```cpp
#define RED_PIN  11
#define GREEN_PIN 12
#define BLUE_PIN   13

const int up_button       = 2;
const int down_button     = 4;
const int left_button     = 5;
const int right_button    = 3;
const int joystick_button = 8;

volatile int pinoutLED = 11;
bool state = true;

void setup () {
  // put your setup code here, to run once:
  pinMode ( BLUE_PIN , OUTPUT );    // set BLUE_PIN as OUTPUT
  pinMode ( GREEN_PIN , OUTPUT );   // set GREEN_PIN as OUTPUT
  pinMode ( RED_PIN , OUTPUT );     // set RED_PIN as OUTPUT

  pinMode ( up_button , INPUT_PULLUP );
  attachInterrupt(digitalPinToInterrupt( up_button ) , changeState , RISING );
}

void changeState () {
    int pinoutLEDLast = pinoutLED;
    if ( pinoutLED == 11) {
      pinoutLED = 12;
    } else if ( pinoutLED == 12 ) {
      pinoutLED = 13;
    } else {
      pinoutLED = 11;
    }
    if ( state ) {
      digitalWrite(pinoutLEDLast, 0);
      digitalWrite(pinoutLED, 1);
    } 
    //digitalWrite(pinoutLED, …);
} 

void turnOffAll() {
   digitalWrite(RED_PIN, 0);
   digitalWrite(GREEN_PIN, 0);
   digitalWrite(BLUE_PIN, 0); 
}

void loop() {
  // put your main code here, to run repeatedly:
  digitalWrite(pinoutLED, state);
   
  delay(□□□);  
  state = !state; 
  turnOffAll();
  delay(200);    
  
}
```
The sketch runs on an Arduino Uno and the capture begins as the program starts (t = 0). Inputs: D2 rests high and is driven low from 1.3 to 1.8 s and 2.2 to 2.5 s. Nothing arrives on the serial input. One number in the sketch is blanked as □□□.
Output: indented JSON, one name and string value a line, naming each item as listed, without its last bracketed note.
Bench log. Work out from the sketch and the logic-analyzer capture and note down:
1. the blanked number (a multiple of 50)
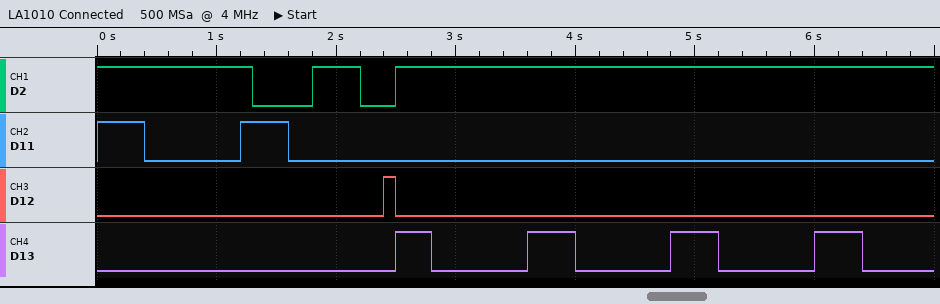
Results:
{
  "the blanked number": "400"
}
